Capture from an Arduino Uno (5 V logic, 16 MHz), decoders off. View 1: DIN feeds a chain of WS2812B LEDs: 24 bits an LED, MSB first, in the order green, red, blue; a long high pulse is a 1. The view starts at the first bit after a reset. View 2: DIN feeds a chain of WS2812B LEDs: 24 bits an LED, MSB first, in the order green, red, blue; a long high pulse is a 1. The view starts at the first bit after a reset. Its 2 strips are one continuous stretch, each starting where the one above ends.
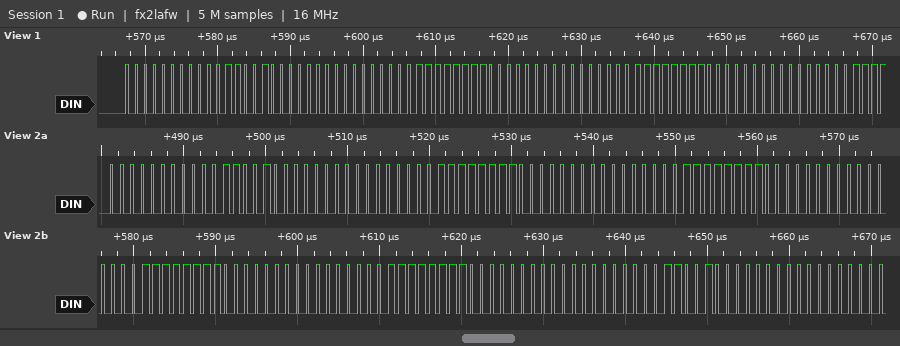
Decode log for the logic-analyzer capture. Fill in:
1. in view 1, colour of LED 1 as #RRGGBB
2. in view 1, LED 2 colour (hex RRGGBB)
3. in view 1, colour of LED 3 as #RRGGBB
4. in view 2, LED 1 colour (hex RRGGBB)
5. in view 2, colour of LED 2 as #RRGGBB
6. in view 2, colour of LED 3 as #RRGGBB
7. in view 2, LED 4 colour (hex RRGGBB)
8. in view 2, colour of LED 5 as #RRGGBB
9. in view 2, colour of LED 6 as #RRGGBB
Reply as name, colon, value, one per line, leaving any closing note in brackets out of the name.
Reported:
in view 1, colour of LED 1 as #RRGGBB: #190000
in view 1, LED 2 colour: #FF0000
in view 1, colour of LED 3 as #RRGGBB: #FF0000
in view 2, LED 1 colour: #190000
in view 2, colour of LED 2 as #RRGGBB: #FF0000
in view 2, colour of LED 3 as #RRGGBB: #FF0000
in view 2, LED 4 colour: #FF0000
in view 2, colour of LED 5 as #RRGGBB: #FF0000
in view 2, colour of LED 6 as #RRGGBB: #190000
